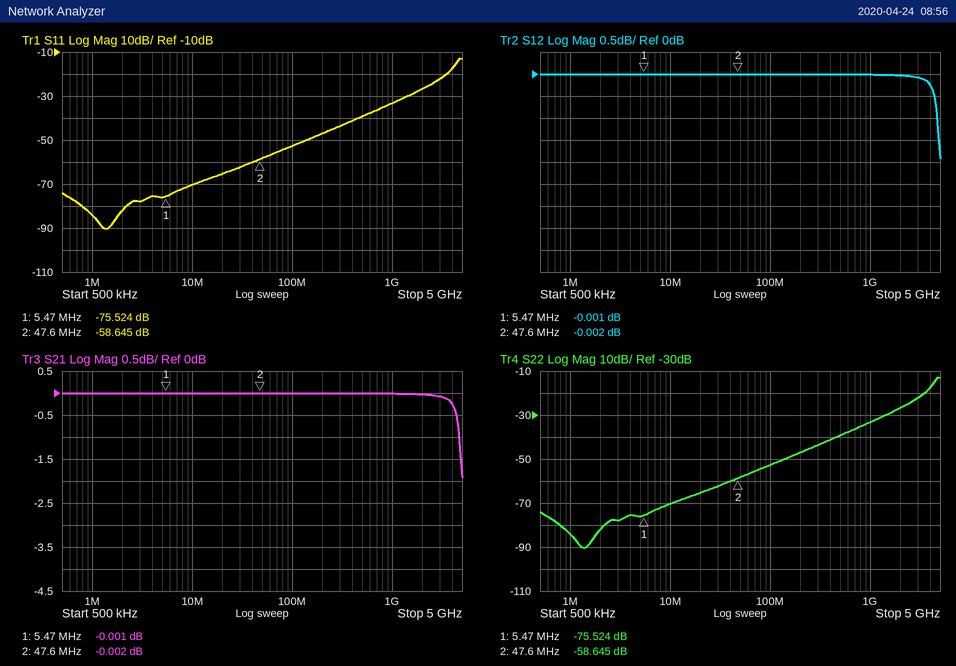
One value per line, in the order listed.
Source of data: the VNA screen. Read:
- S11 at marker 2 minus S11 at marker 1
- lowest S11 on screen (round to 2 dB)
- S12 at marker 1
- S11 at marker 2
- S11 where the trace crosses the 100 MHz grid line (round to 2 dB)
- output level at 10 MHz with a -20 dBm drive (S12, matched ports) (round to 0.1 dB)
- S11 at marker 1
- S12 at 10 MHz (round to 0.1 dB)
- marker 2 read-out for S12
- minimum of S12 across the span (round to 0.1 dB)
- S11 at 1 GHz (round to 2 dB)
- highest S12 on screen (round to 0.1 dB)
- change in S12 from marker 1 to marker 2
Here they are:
16.879 dB
-90 dB
-0.001 dB
-58.645 dB
-52 dB
-20.0 dBm
-75.524 dB
0.0 dB
-0.002 dB
-1.9 dB
-34 dB
0.0 dB
-0.001 dB
